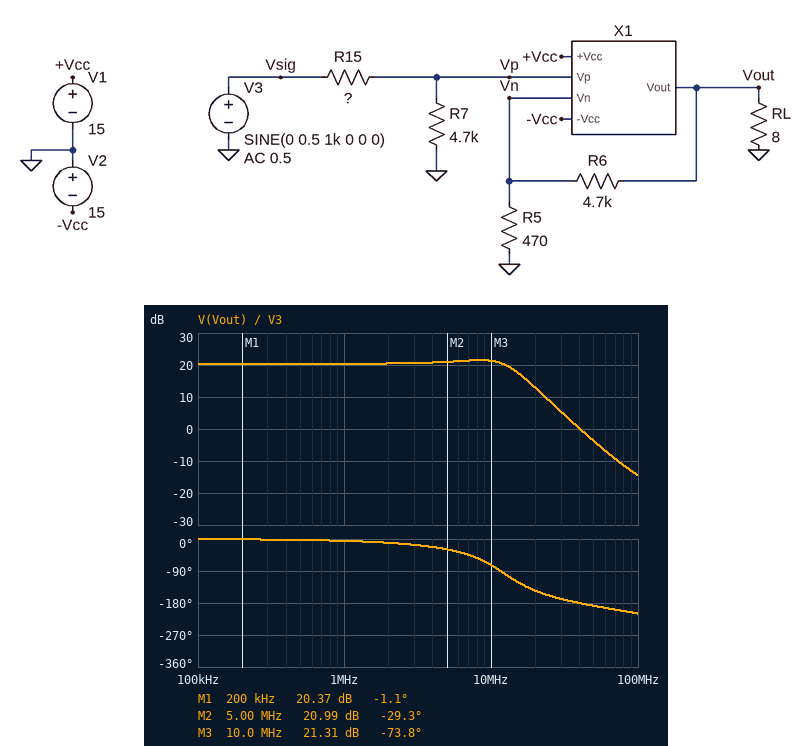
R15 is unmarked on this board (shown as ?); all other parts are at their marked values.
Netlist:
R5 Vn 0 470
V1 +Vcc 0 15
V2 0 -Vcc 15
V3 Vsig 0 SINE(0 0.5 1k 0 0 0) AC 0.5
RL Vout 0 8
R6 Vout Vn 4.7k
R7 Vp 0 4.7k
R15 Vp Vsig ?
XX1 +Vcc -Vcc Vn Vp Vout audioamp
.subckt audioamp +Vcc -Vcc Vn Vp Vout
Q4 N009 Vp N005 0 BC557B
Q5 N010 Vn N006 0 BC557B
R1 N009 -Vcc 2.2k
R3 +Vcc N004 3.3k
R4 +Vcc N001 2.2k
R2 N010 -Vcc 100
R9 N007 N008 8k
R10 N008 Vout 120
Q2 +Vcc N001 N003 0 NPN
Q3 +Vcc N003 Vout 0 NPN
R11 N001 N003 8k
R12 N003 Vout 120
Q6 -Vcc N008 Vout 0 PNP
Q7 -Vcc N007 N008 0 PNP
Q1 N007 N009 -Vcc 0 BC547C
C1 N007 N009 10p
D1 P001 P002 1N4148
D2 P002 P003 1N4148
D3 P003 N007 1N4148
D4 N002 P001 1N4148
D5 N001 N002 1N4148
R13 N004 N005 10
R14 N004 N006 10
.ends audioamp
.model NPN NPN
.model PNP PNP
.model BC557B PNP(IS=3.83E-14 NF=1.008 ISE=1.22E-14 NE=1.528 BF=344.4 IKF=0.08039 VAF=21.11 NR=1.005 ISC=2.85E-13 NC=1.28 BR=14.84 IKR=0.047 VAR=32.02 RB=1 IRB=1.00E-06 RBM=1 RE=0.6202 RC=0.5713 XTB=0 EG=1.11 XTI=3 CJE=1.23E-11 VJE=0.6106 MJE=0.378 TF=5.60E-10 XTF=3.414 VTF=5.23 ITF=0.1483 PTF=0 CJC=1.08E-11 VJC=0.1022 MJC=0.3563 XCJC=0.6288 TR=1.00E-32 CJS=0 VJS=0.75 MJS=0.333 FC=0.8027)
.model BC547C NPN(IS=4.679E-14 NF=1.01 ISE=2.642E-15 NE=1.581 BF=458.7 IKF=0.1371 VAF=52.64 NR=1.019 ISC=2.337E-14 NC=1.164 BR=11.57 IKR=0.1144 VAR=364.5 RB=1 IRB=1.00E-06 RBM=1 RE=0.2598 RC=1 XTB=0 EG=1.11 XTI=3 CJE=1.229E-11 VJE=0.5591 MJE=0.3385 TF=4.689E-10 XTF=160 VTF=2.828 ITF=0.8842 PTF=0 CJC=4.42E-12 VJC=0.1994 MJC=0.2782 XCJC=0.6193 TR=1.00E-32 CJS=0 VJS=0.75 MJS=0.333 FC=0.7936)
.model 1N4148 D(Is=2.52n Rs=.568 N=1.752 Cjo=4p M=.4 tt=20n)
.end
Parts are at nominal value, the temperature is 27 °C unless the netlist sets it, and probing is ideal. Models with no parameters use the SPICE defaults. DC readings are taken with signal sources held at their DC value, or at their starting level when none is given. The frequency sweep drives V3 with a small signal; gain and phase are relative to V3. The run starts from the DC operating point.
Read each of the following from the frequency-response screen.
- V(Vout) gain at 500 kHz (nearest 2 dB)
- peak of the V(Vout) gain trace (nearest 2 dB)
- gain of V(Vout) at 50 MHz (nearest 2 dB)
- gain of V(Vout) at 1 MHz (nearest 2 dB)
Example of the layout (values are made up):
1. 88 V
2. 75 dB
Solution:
1. 20 dB
2. 22 dB
3. -4 dB
4. 20 dB
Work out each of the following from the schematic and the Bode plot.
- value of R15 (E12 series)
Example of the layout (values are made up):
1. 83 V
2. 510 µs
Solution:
1. 270 Ω
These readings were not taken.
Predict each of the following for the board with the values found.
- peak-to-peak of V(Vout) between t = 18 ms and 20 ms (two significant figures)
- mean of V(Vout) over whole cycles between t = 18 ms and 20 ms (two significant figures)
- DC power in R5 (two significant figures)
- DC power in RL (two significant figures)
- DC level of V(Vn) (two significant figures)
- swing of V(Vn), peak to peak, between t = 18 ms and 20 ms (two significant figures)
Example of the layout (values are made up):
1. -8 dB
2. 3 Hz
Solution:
1. 10 V
2. -1.2 V
3. 24 µW
4. 180 mW
5. -110 mV
6. 950 mV
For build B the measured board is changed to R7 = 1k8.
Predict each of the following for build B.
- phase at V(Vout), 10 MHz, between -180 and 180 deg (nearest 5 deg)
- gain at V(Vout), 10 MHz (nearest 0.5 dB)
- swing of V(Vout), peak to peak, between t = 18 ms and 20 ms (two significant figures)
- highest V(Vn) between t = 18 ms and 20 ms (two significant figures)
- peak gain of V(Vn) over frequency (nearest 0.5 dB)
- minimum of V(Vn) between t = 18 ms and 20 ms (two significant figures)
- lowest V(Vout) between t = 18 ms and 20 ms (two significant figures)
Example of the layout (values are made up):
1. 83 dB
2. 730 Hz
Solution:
1. -70 deg
2. 20.5 dB
3. 9.6 V
4. 330 mV
5. -1.0 dB
6. -540 mV
7. -6.0 V
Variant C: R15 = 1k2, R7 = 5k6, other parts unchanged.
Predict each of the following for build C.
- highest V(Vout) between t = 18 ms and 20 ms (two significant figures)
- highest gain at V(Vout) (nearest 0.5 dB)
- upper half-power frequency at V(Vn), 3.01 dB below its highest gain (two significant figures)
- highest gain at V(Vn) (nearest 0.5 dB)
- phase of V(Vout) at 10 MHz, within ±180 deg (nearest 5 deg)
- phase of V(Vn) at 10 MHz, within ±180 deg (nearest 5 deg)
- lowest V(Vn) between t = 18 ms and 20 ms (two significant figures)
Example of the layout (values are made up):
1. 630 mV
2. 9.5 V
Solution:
1. 3.3 V
2. 23.0 dB
3. 8.3 MHz
4. 1.5 dB
5. -140 deg
6. -145 deg
7. -520 mV
